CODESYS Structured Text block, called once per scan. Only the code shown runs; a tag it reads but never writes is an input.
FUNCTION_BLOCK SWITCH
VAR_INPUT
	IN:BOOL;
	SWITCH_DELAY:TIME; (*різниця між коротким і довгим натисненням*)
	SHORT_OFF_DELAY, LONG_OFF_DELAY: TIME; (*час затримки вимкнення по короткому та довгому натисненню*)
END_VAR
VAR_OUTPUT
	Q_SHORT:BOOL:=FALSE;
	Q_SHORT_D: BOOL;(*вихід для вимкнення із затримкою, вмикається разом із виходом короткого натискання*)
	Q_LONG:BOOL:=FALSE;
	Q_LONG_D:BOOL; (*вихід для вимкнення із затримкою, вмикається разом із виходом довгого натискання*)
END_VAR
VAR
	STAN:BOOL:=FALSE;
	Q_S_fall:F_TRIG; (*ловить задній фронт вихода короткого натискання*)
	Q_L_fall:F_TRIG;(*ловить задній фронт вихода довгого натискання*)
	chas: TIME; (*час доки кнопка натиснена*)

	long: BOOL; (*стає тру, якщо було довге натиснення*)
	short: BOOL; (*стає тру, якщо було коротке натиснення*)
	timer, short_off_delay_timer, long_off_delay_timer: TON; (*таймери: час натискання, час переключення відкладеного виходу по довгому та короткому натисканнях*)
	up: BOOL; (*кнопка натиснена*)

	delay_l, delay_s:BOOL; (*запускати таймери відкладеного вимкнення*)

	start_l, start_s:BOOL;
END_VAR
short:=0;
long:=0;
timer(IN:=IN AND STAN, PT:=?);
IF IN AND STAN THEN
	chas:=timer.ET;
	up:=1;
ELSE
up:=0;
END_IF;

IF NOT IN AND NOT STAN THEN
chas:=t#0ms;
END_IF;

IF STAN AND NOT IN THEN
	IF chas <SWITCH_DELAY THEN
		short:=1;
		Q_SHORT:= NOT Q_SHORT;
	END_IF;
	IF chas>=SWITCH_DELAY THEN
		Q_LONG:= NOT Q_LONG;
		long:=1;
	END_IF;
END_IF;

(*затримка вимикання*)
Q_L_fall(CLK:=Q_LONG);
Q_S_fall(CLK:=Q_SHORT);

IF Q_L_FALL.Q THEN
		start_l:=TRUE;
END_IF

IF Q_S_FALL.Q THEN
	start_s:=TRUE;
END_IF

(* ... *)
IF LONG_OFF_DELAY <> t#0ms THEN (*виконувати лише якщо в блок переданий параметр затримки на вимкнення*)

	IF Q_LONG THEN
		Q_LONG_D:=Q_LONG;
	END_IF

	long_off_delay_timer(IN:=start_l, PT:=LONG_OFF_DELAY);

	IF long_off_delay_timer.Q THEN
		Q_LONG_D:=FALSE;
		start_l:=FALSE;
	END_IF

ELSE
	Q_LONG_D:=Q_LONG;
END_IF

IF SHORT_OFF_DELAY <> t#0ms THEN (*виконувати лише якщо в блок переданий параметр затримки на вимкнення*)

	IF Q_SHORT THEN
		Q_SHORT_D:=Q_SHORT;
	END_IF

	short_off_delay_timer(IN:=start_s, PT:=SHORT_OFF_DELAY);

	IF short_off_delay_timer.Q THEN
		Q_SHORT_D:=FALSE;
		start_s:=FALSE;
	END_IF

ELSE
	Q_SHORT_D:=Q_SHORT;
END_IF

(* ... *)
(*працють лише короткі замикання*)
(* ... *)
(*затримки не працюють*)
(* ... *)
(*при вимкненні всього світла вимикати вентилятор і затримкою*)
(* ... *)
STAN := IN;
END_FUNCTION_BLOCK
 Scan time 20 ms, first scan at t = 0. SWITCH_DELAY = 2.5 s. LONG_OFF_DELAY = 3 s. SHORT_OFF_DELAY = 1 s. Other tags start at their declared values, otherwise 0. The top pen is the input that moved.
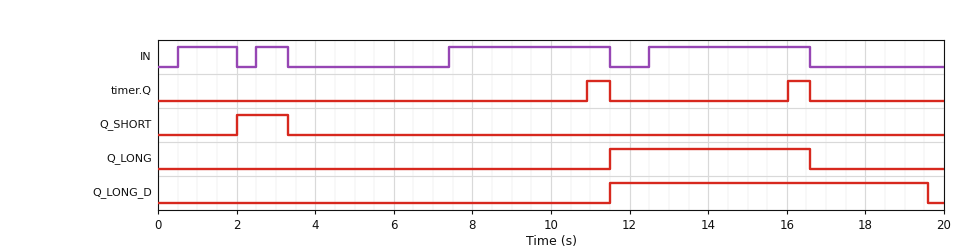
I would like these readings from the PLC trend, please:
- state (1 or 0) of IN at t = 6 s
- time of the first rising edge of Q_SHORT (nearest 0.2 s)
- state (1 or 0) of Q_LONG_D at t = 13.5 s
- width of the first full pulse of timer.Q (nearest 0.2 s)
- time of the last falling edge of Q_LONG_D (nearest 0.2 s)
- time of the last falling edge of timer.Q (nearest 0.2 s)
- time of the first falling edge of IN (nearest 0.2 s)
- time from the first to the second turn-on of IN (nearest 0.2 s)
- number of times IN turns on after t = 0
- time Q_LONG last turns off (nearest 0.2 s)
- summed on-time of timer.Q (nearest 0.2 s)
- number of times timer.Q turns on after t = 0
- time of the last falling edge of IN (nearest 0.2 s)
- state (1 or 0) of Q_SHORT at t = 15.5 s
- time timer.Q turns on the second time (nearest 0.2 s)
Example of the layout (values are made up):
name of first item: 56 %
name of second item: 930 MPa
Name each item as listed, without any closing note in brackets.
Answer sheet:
state (1 or 0) of IN at t = 6 s: 0
time of the first rising edge of Q_SHORT: 2.0 s
state (1 or 0) of Q_LONG_D at t = 13.5 s: 1
width of the first full pulse of timer.Q: 0.6 s
time of the last falling edge of Q_LONG_D: 19.6 s
time of the last falling edge of timer.Q: 16.6 s
time of the first falling edge of IN: 2.0 s
time from the first to the second turn-on of IN: 2.0 s
number of times IN turns on after t = 0: 4
time Q_LONG last turns off: 16.6 s
summed on-time of timer.Q: 1.2 s
number of times timer.Q turns on after t = 0: 2
time of the last falling edge of IN: 16.6 s
state (1 or 0) of Q_SHORT at t = 15.5 s: 0
time timer.Q turns on the second time: 16.0 s
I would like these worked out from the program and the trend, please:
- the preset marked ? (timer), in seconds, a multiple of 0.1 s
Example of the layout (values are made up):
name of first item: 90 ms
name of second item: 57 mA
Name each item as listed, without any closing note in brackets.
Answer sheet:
the preset marked ? (timer), in seconds, a multiple of 0.1 s: 3.5 s
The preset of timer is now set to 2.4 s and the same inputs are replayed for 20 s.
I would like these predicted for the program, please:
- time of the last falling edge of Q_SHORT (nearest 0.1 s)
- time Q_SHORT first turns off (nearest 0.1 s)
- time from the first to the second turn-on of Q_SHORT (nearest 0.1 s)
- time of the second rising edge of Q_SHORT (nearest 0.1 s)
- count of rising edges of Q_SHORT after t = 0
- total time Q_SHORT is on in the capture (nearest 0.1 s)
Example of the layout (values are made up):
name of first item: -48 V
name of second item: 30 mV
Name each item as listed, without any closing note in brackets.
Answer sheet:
time of the last falling edge of Q_SHORT: 16.6 s
time Q_SHORT first turns off: 3.3 s
time from the first to the second turn-on of Q_SHORT: 9.5 s
time of the second rising edge of Q_SHORT: 11.5 s
count of rising edges of Q_SHORT after t = 0: 2
total time Q_SHORT is on in the capture: 6.4 s
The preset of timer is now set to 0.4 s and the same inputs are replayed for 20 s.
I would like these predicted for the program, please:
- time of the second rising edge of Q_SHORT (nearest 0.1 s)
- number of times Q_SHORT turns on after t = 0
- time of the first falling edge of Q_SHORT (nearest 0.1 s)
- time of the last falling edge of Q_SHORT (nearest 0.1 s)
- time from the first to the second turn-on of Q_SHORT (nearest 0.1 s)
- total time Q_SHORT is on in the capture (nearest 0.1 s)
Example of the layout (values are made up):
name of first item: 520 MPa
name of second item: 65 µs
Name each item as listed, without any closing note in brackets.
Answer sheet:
time of the second rising edge of Q_SHORT: 11.5 s
number of times Q_SHORT turns on after t = 0: 2
time of the first falling edge of Q_SHORT: 3.3 s
time of the last falling edge of Q_SHORT: 16.6 s
time from the first to the second turn-on of Q_SHORT: 9.5 s
total time Q_SHORT is on in the capture: 6.4 s
